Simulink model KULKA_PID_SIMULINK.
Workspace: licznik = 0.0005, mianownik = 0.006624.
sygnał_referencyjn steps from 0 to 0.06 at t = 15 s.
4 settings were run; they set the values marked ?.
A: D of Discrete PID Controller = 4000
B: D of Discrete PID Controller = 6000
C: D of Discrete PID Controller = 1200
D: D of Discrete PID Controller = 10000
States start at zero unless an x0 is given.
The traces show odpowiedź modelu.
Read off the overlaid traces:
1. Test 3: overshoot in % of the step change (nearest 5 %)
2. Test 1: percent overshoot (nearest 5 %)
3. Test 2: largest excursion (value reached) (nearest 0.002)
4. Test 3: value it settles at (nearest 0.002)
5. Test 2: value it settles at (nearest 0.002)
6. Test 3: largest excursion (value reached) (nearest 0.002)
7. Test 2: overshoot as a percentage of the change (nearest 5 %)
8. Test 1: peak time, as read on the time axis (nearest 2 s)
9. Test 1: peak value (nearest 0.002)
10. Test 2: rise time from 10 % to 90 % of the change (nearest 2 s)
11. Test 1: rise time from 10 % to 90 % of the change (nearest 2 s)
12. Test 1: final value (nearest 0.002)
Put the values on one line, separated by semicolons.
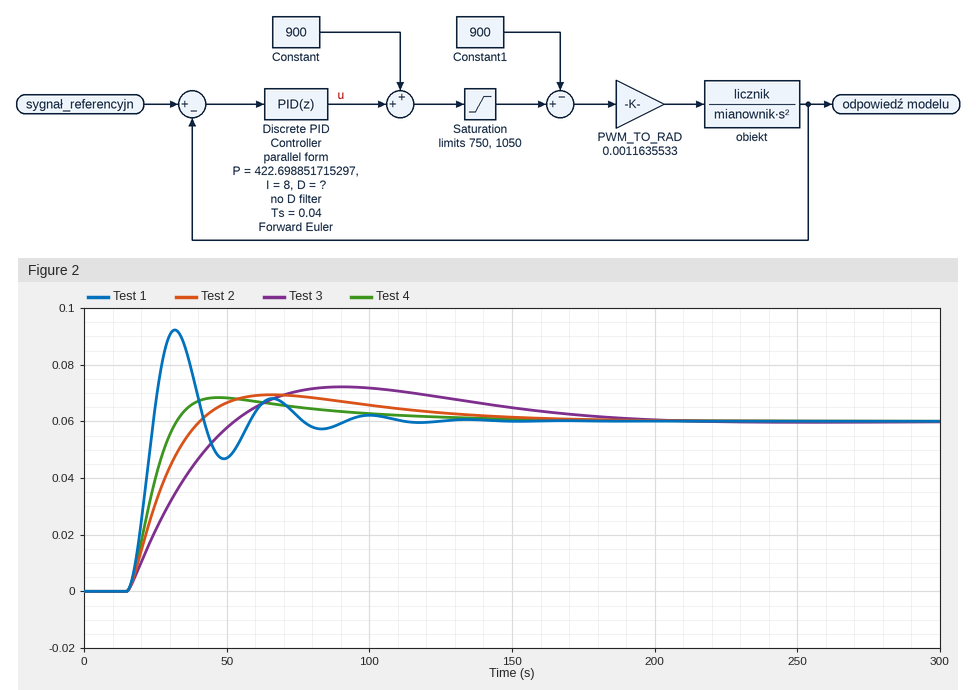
20 %; 55 %; 0.070; 0.060; 0.060; 0.072; 15 %; 32 s; 0.092; 18 s; 6 s; 0.060
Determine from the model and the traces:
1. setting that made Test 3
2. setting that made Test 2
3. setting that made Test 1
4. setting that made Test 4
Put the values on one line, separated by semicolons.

D; B; C; A
